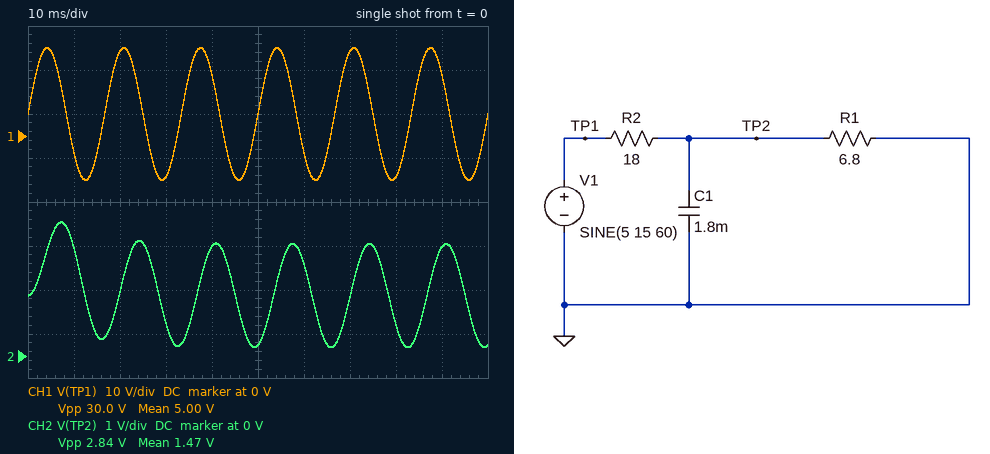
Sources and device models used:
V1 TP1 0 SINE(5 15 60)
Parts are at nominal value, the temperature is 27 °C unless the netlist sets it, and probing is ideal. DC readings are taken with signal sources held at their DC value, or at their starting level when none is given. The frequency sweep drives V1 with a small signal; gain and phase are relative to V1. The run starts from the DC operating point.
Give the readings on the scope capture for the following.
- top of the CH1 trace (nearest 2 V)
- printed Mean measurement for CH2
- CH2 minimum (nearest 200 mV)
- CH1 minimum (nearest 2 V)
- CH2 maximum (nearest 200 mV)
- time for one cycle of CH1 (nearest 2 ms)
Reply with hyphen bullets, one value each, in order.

- 20 V
- 1.47 V
- 200 mV
- -10 V
- 3.0 V
- 16 ms
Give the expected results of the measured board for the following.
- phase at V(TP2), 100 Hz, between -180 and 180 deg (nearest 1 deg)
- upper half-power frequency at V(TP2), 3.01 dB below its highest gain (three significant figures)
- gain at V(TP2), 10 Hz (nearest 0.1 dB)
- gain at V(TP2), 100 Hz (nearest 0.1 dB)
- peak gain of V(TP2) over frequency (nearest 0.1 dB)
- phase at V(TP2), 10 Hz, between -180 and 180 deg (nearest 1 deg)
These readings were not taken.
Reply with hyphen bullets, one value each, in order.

- -80 deg
- 17.9 Hz
- -12.4 dB
- -26.3 dB
- -11.2 dB
- -29 deg
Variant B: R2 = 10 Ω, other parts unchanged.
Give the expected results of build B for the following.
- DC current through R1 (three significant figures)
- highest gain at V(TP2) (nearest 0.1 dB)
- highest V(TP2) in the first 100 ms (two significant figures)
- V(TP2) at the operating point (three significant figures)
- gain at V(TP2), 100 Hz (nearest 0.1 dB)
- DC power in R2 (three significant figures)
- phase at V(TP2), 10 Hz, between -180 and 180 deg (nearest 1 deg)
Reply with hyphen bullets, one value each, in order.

- 298 mA
- -7.9 dB
- 4.8 V
- 2.02 V
- -21.3 dB
- 886 mW
- -25 deg
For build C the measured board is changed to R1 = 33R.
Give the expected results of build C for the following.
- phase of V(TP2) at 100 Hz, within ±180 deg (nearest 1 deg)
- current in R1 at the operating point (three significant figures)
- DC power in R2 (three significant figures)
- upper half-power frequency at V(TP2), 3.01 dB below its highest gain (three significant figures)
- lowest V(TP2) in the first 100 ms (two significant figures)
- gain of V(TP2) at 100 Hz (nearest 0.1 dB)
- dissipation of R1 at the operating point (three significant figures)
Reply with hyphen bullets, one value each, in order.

- -86 deg
- 98.0 mA
- 173 mW
- 7.59 Hz
- 2.0 V
- -26.2 dB
- 317 mW
